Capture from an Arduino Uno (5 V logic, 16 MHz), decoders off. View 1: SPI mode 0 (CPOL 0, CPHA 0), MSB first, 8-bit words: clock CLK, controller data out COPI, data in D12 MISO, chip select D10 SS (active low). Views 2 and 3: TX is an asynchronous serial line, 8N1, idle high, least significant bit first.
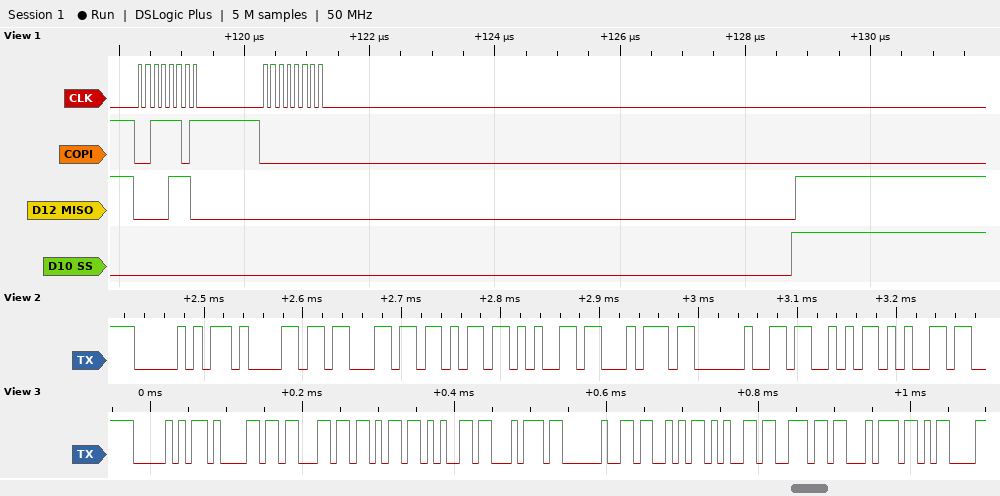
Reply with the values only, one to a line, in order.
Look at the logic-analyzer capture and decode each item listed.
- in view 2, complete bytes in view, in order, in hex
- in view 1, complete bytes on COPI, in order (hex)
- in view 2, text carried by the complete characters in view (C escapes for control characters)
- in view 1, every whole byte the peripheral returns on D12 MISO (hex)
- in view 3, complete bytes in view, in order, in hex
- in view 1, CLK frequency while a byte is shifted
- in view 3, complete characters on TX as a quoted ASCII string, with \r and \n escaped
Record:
50 61 63 6B 65 74 20 53 65
3D 00
"Packet Se"
0E 00
50 61 63 6B 65 74 20 53 65 6E 74 0D
8 MHz
"Packet Sent\r"
